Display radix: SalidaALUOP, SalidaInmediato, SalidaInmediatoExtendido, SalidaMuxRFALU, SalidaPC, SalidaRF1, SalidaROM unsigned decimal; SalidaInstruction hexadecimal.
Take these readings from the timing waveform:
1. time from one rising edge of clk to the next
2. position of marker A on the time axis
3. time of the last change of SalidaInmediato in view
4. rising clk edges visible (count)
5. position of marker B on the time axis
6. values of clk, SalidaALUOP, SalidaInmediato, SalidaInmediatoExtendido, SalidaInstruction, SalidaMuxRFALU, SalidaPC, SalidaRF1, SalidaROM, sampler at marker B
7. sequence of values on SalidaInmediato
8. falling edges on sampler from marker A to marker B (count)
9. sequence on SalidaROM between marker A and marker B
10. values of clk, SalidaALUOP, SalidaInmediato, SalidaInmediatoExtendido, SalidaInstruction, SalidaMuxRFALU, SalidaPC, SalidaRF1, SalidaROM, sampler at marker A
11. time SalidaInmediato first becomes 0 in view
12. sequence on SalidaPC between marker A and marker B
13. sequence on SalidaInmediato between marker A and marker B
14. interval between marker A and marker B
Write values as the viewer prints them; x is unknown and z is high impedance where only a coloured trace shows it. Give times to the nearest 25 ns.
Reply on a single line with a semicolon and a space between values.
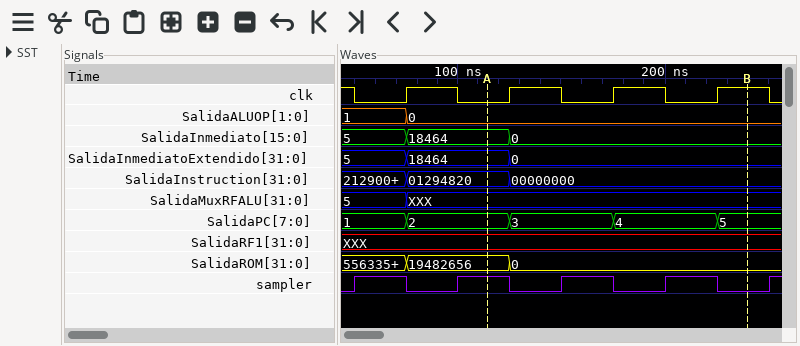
50 ns; 125 ns; 125 ns; 4; 250 ns; clk=1, SalidaALUOP=0, SalidaInmediato=0, SalidaInmediatoExtendido=0, SalidaInstruction=00000000, SalidaMuxRFALU=XXX, SalidaPC=5, SalidaRF1=XXX, SalidaROM=0, sampler=0; 5, 18464, 0; 3; 19482656, 0; clk=0, SalidaALUOP=0, SalidaInmediato=18464, SalidaInmediatoExtendido=18464, SalidaInstruction=01294820, SalidaMuxRFALU=XXX, SalidaPC=2, SalidaRF1=XXX, SalidaROM=19482656, sampler=1; 125 ns; 2, 3, 4, 5; 18464, 0; 125 ns
